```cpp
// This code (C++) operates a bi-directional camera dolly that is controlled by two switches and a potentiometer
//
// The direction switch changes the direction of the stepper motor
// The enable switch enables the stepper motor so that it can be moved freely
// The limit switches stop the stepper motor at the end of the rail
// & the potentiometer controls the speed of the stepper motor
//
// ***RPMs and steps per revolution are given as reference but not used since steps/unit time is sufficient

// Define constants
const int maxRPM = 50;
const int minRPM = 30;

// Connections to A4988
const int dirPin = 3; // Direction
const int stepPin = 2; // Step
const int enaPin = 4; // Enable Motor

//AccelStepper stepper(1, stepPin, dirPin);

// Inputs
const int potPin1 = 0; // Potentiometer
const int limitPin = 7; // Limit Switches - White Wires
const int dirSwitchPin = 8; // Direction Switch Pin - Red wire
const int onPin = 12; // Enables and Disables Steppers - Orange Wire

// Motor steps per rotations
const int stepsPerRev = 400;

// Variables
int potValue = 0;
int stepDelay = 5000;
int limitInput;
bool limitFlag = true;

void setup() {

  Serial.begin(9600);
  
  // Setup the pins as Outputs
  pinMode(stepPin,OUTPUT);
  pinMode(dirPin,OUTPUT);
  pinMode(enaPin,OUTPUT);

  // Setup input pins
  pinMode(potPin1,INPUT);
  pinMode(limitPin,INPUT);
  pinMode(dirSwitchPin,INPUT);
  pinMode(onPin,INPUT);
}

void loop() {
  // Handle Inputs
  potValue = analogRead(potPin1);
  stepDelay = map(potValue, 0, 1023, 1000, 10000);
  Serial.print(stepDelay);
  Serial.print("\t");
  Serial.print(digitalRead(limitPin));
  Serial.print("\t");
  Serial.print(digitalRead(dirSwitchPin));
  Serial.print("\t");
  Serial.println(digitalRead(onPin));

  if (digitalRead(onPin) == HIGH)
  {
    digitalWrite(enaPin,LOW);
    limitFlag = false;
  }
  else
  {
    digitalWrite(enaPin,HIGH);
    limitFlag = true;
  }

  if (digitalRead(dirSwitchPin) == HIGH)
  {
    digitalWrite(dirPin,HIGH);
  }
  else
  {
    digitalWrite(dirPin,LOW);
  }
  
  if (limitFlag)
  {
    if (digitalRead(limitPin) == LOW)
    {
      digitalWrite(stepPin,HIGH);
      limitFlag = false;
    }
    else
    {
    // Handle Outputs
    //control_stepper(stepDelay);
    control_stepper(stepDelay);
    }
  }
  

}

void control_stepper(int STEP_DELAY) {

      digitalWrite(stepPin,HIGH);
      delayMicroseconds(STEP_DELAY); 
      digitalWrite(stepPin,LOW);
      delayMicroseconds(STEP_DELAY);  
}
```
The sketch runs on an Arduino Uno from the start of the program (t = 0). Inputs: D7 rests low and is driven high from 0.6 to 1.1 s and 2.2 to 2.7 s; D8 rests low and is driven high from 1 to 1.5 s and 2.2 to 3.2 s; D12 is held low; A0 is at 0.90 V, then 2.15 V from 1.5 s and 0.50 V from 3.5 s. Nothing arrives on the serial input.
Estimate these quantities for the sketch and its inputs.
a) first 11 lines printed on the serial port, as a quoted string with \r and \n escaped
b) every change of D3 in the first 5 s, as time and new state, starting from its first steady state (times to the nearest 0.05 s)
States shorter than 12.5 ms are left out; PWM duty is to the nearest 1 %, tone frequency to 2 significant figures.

"2618\t0\t0\t0\r\n2618\t0\t0\t0\r\n2618\t0\t0\t0\r\n2618\t0\t0\t0\r\n2618\t0\t0\t0\r\n2618\t0\t0\t0\r\n2618\t0\t0\t0\r\n2618\t0\t0\t0\r\n2618\t0\t0\t0\r\n2618\t0\t0\t0\r\n2618\t0\t0\t0\r\n"
0 s low; 1 s high; 1.5 s low; 2.2 s high; 3.2 s low
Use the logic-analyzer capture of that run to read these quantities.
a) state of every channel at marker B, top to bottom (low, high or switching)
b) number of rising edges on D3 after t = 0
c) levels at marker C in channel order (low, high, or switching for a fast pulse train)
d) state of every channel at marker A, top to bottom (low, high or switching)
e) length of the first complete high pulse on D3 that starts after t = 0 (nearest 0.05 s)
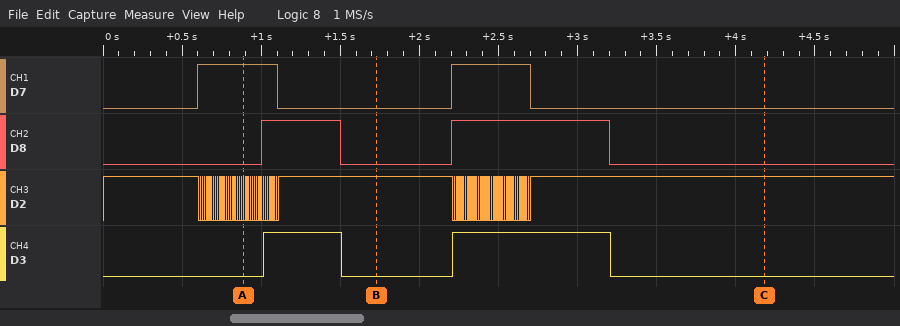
D7 low, D8 low, D2 high, D3 low
2
D7 low, D8 low, D2 high, D3 low
D7 high, D8 low, D2 switching, D3 low
0.50 s
